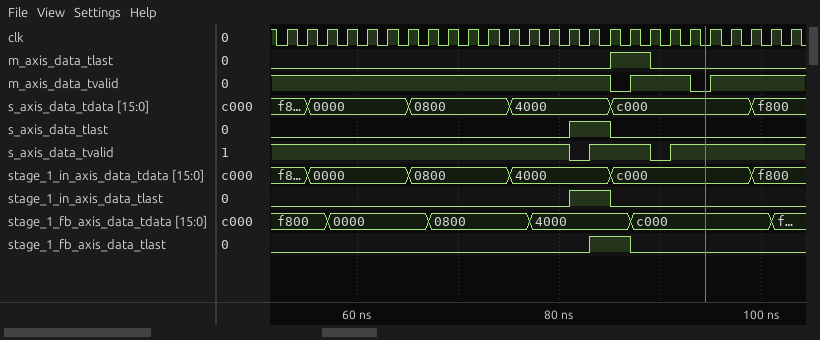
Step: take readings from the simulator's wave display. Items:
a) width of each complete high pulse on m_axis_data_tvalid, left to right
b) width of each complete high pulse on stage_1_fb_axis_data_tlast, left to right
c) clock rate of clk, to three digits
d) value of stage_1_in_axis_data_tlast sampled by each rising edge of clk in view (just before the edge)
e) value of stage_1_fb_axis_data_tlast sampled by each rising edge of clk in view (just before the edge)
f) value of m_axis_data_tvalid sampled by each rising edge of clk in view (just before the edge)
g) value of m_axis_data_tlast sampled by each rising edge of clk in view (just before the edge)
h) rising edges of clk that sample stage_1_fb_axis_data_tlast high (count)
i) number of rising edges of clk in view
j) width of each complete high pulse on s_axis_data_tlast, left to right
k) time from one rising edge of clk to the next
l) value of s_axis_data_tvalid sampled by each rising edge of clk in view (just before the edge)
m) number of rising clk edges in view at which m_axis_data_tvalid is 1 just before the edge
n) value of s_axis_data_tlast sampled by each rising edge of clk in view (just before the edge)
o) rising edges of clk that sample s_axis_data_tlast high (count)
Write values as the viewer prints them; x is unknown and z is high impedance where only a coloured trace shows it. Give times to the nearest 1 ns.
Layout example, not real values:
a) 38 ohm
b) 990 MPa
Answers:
a) 6 ns
b) 4 ns
c) 500 MHz
d) 0 0 0 0 0 0 0 0 0 0 0 0 0 0 0 1 1 0 0 0 0 0 0 0 0 0
e) 0 0 0 0 0 0 0 0 0 0 0 0 0 0 0 0 1 1 0 0 0 0 0 0 0 0
f) 1 1 1 1 1 1 1 1 1 1 1 1 1 1 1 1 1 0 1 1 1 0 1 1 1 1
g) 0 0 0 0 0 0 0 0 0 0 0 0 0 0 0 0 0 1 1 0 0 0 0 0 0 0
h) 2
i) 26
j) 4 ns
k) 2 ns
l) 1 1 1 1 1 1 1 1 1 1 1 1 1 1 1 0 1 1 1 0 1 1 1 1 1 1
m) 24
n) 0 0 0 0 0 0 0 0 0 0 0 0 0 0 0 1 1 0 0 0 0 0 0 0 0 0
o) 2
